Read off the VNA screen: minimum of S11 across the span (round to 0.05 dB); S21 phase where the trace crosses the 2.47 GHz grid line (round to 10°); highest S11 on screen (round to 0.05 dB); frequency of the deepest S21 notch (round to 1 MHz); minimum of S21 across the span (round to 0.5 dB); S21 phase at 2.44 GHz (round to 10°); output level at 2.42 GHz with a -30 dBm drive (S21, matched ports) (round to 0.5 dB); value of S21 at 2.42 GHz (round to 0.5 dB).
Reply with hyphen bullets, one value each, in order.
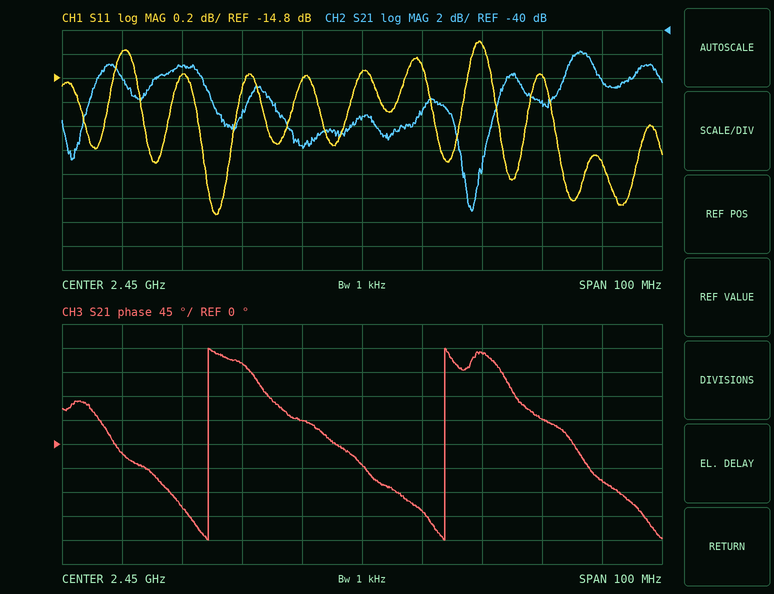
- -15.95 dB
- 170°
- -14.50 dB
- 2.468 GHz
- -55.0 dB
- 40°
- -73.0 dBm
- -43.0 dB
